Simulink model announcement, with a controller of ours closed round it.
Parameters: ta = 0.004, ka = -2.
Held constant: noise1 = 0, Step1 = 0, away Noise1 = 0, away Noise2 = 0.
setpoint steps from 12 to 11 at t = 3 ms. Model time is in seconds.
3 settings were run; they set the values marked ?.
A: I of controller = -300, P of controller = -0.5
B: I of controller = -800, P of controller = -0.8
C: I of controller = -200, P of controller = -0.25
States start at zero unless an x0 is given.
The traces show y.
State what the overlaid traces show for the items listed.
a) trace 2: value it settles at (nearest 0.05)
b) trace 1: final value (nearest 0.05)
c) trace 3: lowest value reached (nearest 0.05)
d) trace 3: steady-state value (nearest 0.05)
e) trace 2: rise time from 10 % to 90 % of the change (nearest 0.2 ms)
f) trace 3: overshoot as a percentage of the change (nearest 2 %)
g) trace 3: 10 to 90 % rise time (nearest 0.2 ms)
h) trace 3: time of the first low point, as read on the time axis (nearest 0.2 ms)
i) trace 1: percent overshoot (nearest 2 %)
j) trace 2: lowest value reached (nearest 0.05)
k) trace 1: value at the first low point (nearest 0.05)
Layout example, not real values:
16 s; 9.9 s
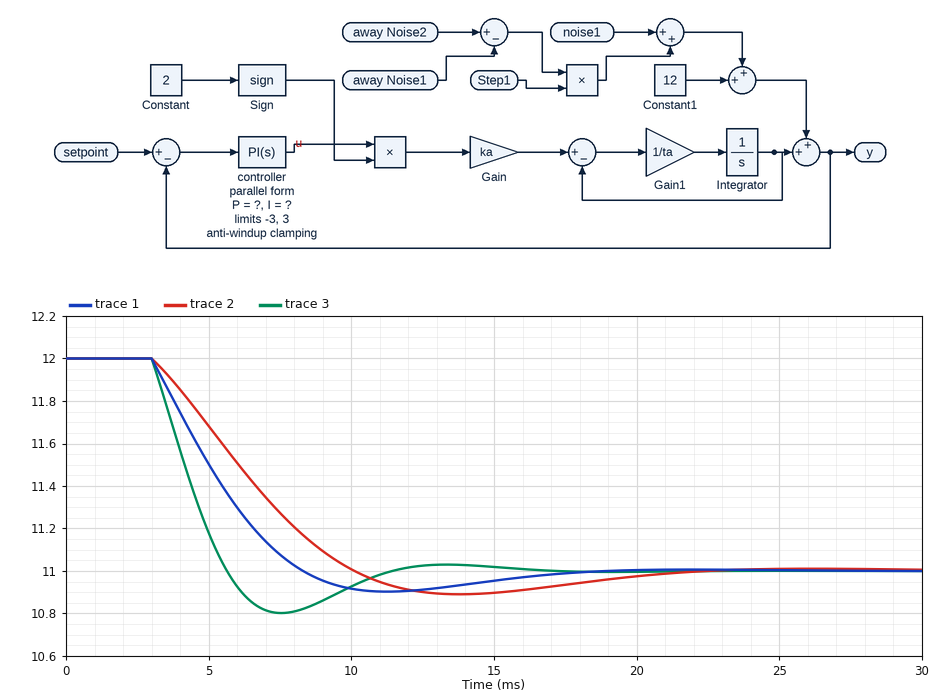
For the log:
11.00; 11.00; 10.80; 11.00; 5.2 ms; 20 %; 2.0 ms; 7.6 ms; 10 %; 10.90; 10.90
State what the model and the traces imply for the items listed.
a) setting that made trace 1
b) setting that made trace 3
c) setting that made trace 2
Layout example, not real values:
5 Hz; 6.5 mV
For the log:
A; B; C
